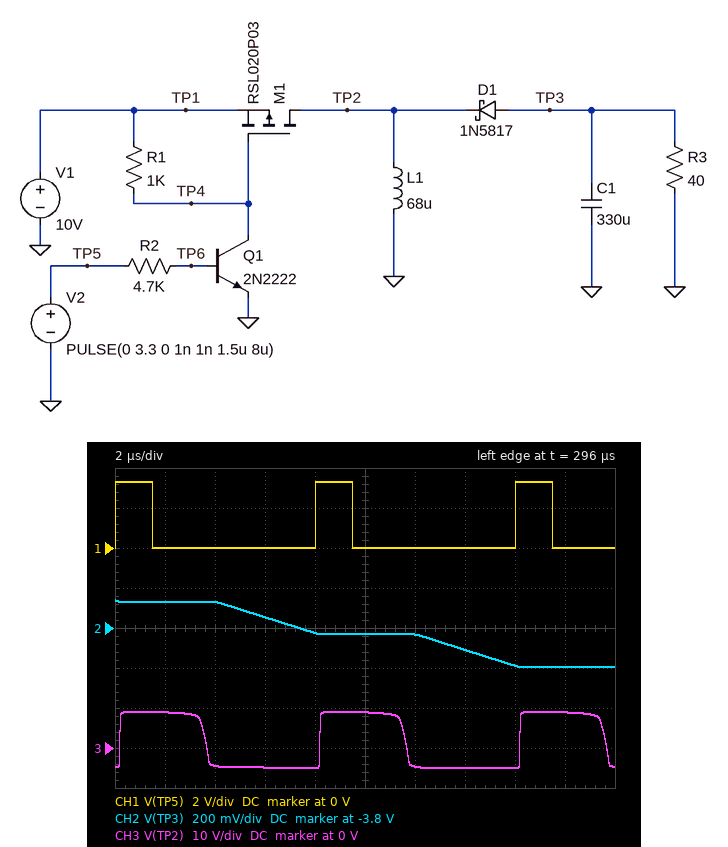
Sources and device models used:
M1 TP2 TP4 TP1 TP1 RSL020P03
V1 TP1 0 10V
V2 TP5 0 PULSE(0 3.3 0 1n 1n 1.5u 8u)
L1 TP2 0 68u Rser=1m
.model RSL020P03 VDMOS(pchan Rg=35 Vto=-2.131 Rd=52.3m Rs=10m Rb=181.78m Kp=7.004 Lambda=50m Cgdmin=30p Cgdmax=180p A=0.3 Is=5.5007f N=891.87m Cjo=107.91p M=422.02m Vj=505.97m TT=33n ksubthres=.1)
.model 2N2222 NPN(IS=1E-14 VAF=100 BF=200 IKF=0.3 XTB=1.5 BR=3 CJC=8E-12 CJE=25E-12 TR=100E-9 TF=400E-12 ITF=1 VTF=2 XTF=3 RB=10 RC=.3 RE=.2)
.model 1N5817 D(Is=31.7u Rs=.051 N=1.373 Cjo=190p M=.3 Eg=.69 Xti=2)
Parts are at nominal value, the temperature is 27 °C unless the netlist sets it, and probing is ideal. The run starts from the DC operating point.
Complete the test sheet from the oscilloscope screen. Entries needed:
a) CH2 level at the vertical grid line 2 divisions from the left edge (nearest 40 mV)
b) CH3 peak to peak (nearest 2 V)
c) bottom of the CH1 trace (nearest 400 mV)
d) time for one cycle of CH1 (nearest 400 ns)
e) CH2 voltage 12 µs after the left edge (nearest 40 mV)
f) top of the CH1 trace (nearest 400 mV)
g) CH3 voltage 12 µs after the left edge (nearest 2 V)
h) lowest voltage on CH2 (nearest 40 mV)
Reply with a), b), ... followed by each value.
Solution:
a) -3.68 V
b) 14 V
c) 0 V
d) 8.0 µs
e) -3.84 V
f) 3.2 V
g) -4 V
h) -4.00 V
